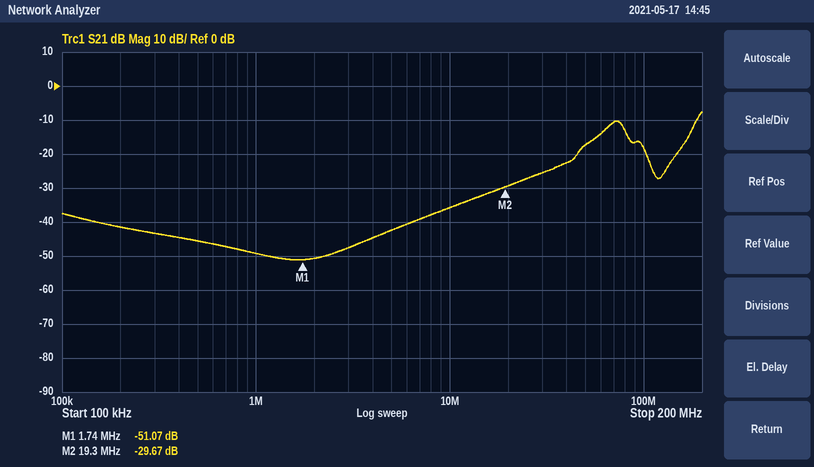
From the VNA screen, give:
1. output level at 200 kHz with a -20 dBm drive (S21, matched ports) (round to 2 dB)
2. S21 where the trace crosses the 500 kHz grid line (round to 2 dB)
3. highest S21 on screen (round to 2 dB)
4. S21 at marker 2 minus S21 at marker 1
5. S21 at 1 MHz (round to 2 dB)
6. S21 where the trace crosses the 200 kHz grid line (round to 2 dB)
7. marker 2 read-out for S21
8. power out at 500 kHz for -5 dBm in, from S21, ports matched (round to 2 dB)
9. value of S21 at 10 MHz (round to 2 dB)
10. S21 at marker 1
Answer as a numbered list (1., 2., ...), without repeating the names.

1. -62 dBm
2. -46 dB
3. -8 dB
4. 21.40 dB
5. -50 dB
6. -42 dB
7. -29.67 dB
8. -50 dBm
9. -36 dB
10. -51.07 dB
